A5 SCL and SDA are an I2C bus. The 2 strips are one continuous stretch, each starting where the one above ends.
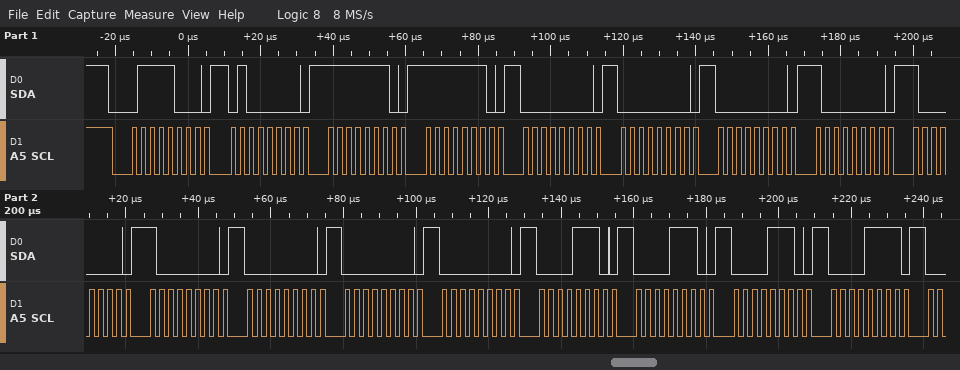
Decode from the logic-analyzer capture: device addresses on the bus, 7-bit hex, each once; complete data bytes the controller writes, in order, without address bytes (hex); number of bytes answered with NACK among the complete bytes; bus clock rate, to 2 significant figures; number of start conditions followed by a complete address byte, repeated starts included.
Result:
0x3C
40 FE FE 00 00 00 80 80 80 00 00 00 0E 0E 0E 0F
0
400 kHz
1
